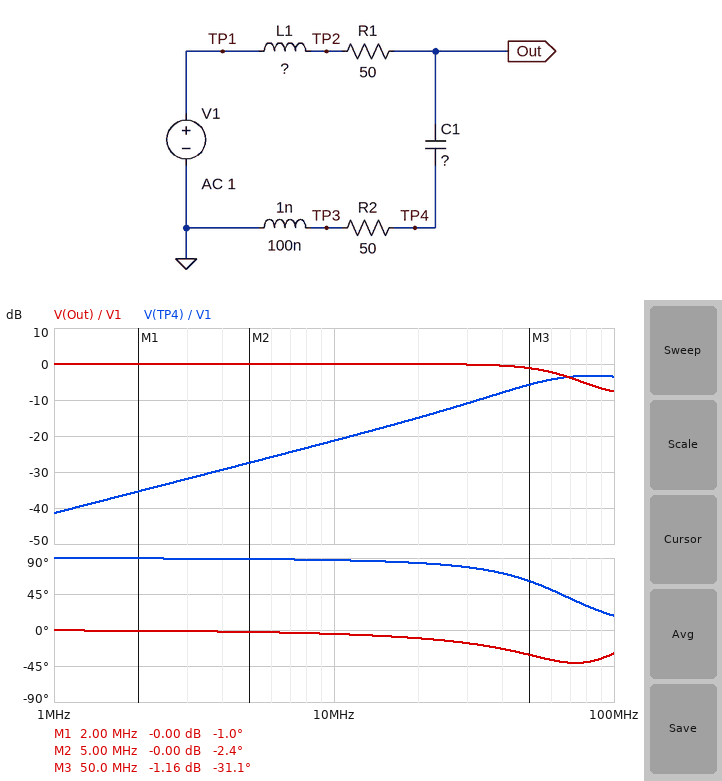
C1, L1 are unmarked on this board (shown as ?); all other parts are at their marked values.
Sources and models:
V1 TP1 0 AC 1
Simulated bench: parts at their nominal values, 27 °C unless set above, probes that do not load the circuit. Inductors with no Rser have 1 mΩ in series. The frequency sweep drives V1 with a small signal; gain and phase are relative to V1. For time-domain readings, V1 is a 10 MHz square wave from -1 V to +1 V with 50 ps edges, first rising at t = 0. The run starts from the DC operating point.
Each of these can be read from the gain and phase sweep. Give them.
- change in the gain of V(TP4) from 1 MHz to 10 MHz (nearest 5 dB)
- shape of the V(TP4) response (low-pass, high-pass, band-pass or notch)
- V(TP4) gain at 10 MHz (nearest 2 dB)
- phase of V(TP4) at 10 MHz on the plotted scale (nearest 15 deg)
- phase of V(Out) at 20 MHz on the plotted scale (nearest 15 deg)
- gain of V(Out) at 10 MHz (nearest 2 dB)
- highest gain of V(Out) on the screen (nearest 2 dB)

20 dB
high-pass
-22 dB
90 deg
-15 deg
0 dB
0 dB
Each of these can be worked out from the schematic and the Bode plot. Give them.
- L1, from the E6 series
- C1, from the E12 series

100 nH
27 pF
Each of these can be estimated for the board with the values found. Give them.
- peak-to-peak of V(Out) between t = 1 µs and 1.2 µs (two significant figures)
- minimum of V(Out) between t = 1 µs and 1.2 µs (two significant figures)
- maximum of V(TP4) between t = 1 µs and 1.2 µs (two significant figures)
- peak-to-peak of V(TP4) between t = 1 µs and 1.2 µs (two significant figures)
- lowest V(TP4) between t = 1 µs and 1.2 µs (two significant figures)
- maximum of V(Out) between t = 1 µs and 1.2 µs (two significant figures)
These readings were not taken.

2.2 V
-1.1 V
1.0 V
2.0 V
-1.0 V
1.1 V
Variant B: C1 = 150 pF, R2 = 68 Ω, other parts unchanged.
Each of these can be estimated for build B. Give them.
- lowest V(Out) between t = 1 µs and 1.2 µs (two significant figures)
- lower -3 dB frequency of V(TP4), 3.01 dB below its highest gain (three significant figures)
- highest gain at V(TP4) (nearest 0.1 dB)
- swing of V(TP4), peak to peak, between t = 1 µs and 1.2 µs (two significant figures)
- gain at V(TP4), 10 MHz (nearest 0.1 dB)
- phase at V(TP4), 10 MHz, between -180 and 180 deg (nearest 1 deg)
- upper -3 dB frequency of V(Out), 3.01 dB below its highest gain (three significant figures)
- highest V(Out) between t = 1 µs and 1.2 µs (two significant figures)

-960 mV
8.88 MHz
-4.4 dB
2.0 V
-6.9 dB
44 deg
15.2 MHz
960 mV
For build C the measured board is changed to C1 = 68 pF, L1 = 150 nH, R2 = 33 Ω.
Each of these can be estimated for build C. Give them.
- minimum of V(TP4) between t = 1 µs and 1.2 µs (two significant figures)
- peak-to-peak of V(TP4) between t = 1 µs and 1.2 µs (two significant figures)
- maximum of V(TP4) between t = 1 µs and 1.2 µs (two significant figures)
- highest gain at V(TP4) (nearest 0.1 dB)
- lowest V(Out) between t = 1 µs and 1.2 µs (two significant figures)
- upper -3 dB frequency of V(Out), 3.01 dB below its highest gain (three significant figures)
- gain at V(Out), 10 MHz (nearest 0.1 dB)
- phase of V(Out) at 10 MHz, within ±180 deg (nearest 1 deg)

-800 mV
1.6 V
800 mV
-5.8 dB
-1.1 V
32.9 MHz
-0.1 dB
-13 deg
